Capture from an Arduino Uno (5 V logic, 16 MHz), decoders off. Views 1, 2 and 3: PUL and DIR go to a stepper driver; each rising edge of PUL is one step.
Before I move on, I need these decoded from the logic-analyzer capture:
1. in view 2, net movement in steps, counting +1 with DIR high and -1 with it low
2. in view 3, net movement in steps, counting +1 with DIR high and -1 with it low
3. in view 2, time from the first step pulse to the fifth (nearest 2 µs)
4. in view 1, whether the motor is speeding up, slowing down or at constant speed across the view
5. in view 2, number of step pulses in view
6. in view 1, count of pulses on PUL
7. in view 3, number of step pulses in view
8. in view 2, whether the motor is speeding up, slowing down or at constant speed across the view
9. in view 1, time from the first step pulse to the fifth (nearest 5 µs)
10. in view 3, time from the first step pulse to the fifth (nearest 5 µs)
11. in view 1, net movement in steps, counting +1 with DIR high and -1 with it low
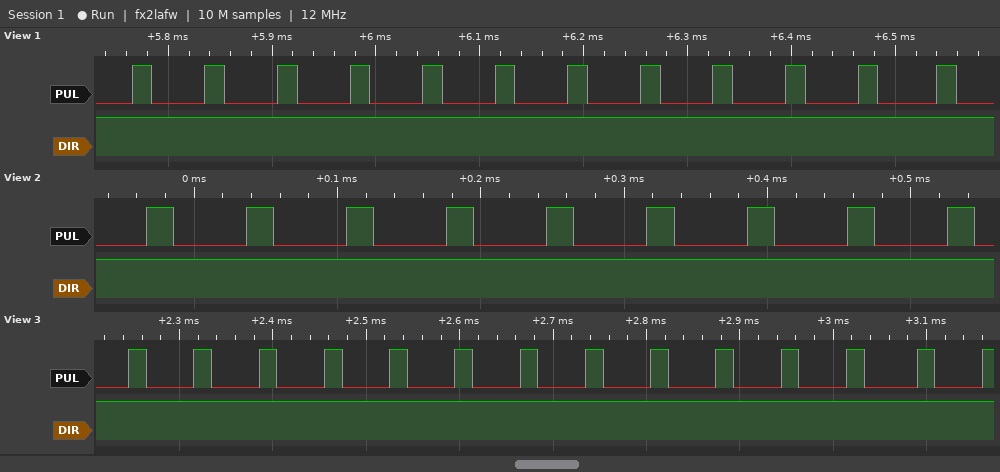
+9
+14
280 µs
slowing down
9
12
14
constant speed
280 µs
280 µs
+12
